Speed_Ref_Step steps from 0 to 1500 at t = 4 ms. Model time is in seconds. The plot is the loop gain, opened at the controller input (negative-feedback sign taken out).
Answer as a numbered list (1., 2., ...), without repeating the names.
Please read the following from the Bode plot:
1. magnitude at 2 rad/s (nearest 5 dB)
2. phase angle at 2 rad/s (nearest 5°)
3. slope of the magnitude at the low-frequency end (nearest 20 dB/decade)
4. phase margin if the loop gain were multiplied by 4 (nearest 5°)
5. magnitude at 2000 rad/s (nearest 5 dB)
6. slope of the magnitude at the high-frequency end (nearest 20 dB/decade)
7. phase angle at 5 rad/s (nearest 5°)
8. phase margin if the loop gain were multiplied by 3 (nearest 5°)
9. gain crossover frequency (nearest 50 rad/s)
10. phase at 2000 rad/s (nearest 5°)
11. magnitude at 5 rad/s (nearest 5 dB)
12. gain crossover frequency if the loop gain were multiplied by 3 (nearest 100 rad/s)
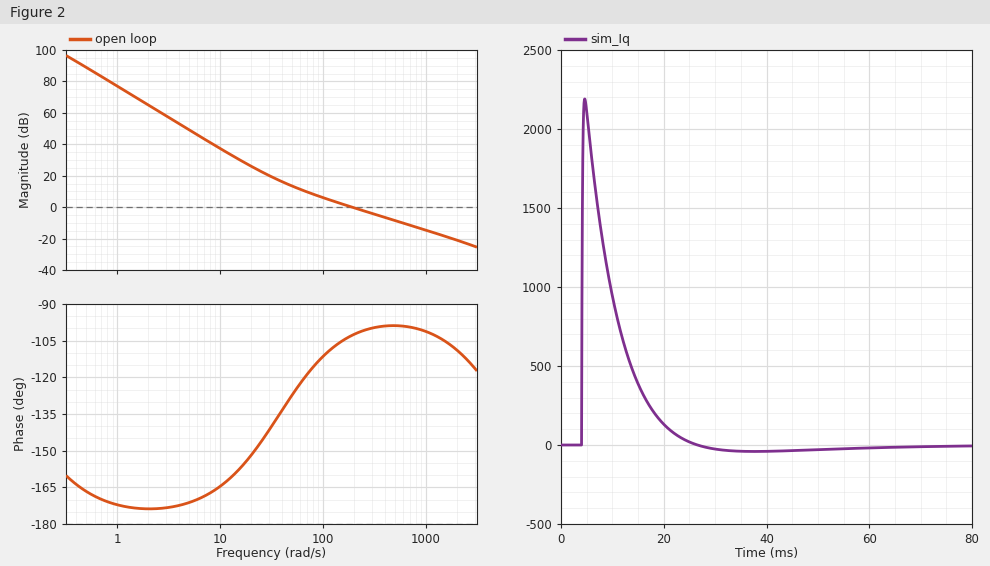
1. 65 dB
2. -175°
3. -40 dB/decade
4. 80°
5. -20 dB
6. -20 dB/decade
7. -170°
8. 80°
9. 200 rad/s
10. -110°
11. 50 dB
12. 600 rad/s
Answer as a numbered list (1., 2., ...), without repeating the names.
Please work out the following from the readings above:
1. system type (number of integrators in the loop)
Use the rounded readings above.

1. 2
